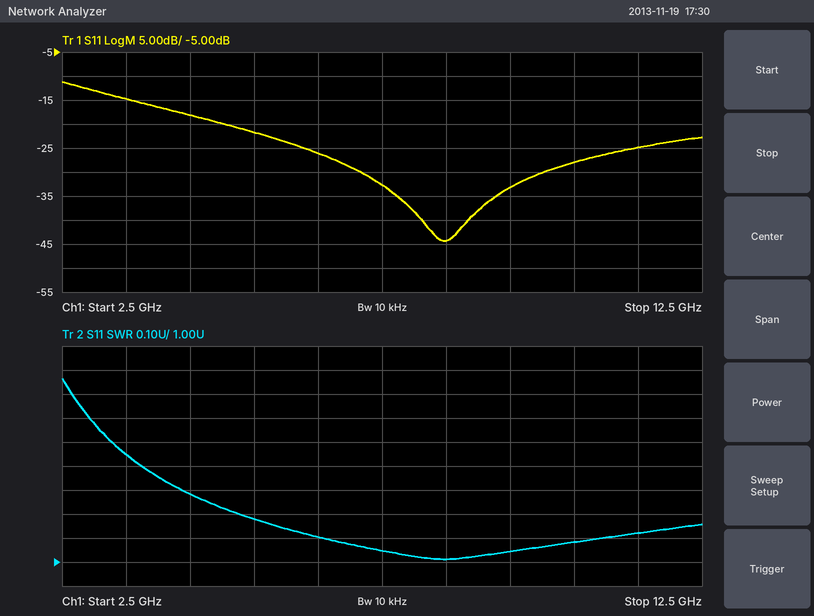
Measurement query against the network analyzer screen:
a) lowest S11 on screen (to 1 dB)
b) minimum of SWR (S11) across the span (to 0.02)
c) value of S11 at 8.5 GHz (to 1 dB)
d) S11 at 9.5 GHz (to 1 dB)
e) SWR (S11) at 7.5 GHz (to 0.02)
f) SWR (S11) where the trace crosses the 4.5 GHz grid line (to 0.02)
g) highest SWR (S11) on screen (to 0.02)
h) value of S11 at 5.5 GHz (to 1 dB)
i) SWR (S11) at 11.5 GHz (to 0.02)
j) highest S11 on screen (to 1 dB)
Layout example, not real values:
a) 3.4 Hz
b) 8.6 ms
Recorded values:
a) -44 dB
b) 1.02
c) -44 dB
d) -33 dB
e) 1.04
f) 1.28
g) 1.76
h) -22 dB
i) 1.12
j) -11 dB
